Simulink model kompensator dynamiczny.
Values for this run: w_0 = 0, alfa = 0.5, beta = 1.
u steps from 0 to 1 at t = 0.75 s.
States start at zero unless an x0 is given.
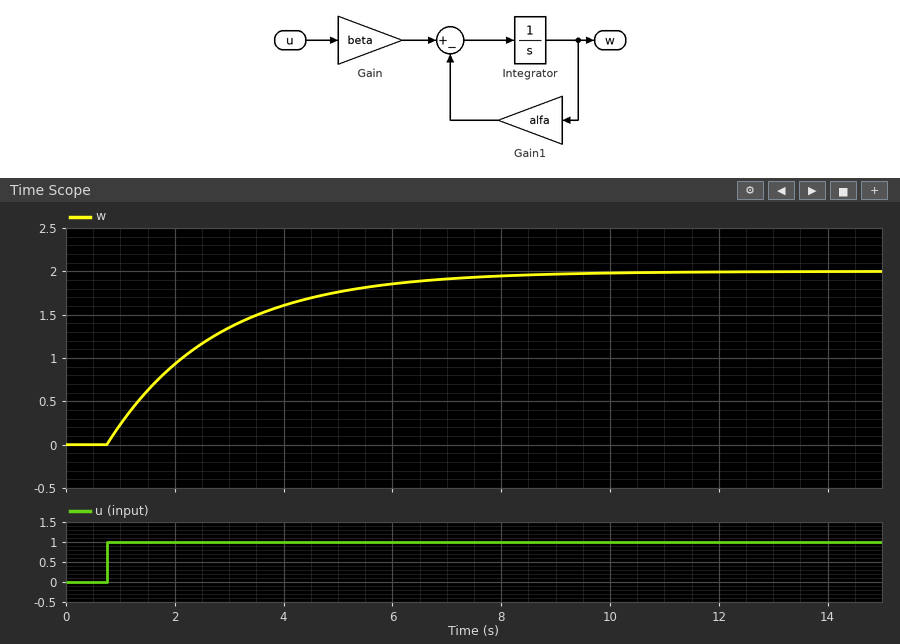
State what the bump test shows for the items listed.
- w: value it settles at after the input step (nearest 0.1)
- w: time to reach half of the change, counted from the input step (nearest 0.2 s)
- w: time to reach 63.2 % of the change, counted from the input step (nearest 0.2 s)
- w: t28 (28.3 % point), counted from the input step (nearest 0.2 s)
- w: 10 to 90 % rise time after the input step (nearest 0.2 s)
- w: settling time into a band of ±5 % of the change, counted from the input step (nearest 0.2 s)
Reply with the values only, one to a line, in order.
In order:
2.0
1.4 s
2.0 s
0.6 s
4.4 s
6.0 s
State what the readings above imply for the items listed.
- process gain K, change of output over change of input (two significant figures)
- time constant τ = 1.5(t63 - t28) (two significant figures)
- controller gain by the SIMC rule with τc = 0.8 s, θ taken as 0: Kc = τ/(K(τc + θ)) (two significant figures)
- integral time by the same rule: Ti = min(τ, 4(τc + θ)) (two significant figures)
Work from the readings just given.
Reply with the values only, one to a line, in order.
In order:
2.0
2.1 s
1.3
2.1 s
